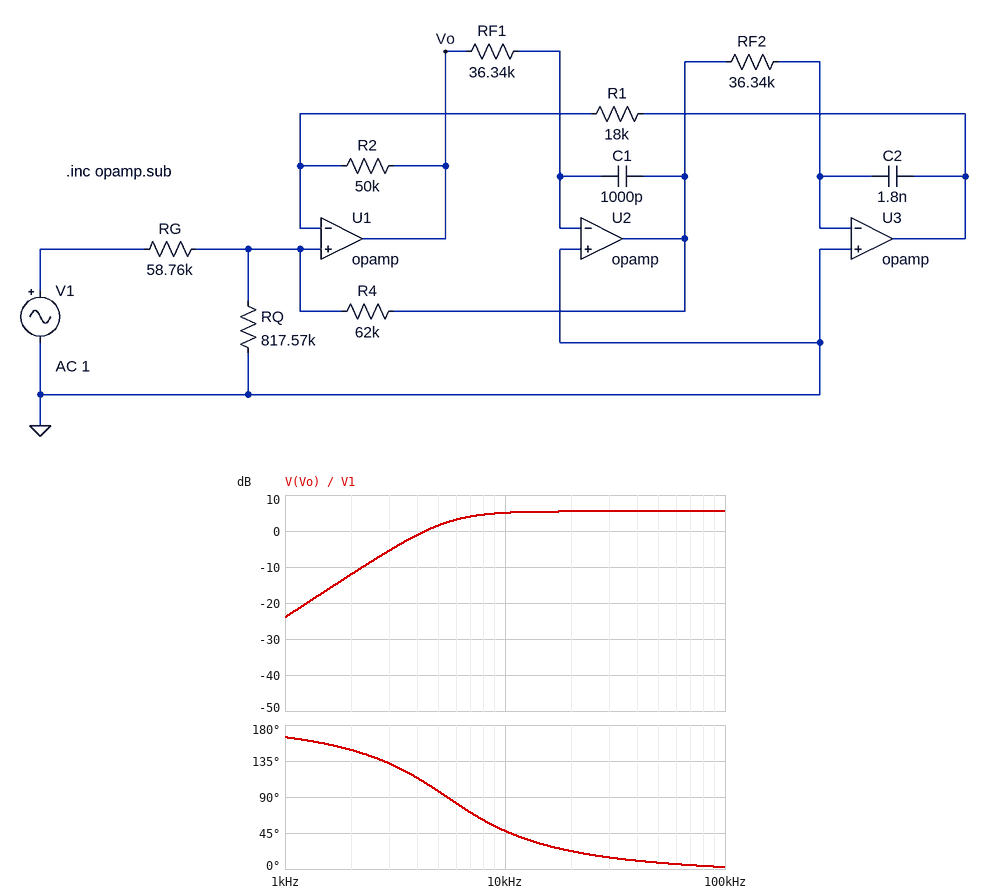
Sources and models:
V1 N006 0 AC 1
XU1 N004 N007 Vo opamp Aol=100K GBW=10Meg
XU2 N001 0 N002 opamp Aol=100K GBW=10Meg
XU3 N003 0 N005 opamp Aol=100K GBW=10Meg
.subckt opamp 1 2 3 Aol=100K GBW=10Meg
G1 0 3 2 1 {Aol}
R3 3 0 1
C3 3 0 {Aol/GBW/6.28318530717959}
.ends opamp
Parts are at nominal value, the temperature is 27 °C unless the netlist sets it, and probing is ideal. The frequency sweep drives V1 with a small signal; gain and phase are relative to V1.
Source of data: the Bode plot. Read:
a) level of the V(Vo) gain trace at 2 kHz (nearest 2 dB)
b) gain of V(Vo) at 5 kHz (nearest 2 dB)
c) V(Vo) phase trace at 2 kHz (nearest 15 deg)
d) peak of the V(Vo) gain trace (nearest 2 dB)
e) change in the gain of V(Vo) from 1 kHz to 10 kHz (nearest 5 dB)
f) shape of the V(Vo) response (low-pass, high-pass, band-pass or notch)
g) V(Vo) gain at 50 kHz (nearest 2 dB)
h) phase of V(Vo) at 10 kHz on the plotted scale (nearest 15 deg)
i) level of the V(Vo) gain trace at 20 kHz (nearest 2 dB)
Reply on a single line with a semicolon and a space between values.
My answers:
-12 dB; 2 dB; 150 deg; 6 dB; 30 dB; high-pass; 6 dB; 45 deg; 6 dB
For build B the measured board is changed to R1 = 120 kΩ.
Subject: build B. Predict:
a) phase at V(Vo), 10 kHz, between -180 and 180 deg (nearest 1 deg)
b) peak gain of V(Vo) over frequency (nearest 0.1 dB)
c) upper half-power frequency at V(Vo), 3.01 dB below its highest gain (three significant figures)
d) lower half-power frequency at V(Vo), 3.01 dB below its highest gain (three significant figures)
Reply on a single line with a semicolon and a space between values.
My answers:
17 deg; -3.1 dB; 7.04 MHz; 2.06 kHz
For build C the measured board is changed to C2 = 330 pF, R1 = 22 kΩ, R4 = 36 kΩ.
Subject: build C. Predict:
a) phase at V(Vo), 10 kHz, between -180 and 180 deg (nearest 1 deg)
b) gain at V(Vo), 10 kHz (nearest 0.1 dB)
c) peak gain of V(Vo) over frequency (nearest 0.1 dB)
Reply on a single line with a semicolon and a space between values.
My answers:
110 deg; 2.4 dB; 4.9 dB
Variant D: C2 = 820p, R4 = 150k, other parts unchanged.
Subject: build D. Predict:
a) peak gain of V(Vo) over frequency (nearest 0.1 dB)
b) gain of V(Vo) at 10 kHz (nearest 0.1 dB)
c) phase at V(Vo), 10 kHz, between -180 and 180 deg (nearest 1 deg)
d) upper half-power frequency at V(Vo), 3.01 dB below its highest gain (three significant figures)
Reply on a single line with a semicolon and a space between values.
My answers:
13.9 dB; 13.3 dB; 51 deg; 14.1 kHz
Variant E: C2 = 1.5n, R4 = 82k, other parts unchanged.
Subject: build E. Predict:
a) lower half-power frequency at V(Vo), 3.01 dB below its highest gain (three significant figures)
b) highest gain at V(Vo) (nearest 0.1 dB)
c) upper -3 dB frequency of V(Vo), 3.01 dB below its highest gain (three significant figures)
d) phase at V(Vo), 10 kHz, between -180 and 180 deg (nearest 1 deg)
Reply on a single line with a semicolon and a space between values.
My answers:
5.22 kHz; 7.2 dB; 2.22 MHz; 46 deg
